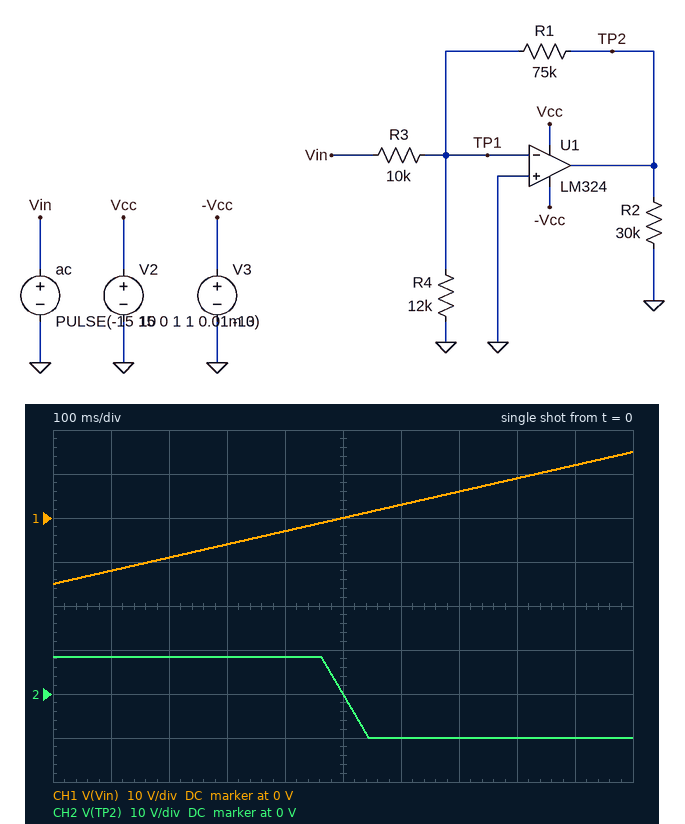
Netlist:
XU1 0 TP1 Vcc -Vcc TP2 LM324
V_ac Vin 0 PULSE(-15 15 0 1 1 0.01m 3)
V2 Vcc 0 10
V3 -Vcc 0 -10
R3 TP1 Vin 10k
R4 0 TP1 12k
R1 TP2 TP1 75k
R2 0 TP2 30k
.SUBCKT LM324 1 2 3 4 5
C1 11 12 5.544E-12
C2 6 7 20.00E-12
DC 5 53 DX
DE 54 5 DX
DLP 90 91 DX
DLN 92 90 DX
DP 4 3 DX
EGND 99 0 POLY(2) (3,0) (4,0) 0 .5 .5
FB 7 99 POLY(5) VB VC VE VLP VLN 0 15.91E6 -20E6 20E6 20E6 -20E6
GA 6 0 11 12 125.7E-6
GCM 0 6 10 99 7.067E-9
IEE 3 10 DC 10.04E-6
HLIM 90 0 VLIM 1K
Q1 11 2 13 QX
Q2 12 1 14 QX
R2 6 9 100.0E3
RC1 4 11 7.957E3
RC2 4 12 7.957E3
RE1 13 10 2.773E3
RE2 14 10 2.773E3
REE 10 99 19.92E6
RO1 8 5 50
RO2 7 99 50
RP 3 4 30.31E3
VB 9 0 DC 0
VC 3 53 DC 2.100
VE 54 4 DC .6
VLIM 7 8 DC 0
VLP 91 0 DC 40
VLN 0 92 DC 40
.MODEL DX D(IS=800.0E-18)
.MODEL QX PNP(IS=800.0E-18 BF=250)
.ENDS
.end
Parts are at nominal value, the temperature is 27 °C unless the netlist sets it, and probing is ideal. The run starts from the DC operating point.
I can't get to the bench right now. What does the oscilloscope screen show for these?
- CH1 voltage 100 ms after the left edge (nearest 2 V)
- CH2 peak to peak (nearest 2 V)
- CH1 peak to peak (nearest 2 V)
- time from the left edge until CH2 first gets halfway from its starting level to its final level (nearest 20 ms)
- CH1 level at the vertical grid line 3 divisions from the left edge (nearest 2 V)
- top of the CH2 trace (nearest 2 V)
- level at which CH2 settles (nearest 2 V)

-12 V
18 V
30 V
500 ms
-6 V
8 V
-10 V
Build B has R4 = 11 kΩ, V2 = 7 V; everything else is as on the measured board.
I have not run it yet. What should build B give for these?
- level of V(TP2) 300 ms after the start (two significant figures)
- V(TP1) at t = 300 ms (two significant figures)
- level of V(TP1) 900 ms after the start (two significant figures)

5.5 V
-2.6 V
5.2 V
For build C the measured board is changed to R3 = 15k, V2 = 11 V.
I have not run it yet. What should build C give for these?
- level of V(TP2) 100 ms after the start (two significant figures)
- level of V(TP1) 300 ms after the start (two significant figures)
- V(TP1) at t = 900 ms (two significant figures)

9.5 V
-1.7 V
4.1 V
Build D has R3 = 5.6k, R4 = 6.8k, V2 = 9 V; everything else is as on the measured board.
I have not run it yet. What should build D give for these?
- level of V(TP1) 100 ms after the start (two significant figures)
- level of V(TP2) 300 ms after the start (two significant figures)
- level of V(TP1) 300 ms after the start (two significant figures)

-6.0 V
7.5 V
-2.9 V
